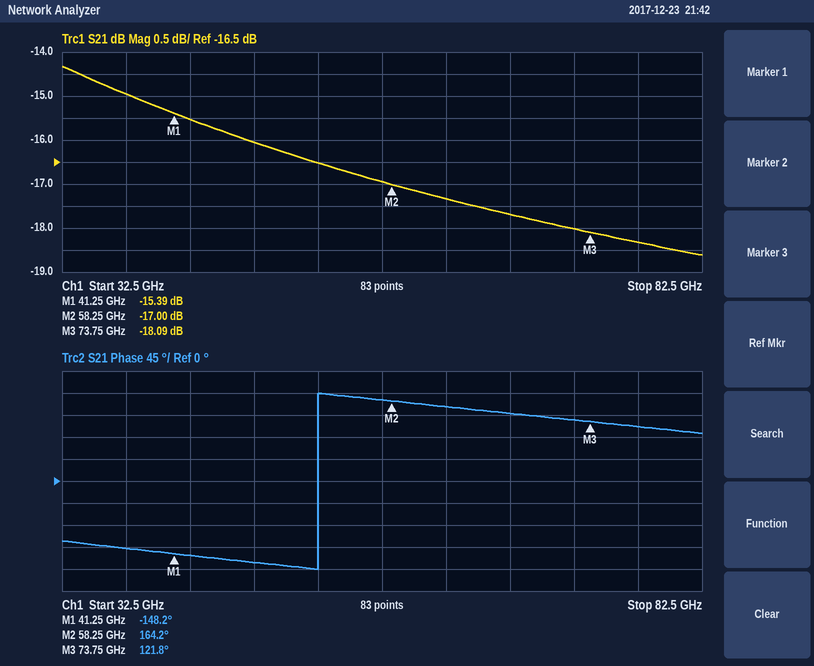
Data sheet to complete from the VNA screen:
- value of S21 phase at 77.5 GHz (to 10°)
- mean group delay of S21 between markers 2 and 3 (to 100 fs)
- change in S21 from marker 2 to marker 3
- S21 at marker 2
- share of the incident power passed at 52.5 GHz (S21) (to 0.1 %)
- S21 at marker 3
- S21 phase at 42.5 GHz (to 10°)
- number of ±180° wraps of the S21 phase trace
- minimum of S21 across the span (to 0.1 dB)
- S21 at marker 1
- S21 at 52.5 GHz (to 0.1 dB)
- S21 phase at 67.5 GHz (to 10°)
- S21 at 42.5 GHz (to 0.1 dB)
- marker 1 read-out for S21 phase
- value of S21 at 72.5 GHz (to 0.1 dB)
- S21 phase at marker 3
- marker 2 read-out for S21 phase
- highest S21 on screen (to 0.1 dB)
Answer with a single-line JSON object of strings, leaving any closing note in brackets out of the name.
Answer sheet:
{"value of S21 phase at 77.5 GHz": "110°", "mean group delay of S21 between markers 2 and 3": "7.6 ps", "change in S21 from marker 2 to marker 3": "-1.09 dB", "S21 at marker 2": "-17.00 dB", "share of the incident power passed at 52.5 GHz (S21)": "2.2 %", "S21 at marker 3": "-18.09 dB", "S21 phase at 42.5 GHz": "-150°", "number of ±180° wraps of the S21 phase trace": "1", "minimum of S21 across the span": "-18.6 dB", "S21 at marker 1": "-15.39 dB", "S21 at 52.5 GHz": "-16.5 dB", "S21 phase at 67.5 GHz": "140°", "S21 at 42.5 GHz": "-15.5 dB", "marker 1 read-out for S21 phase": "-148.2°", "value of S21 at 72.5 GHz": "-18.0 dB", "S21 phase at marker 3": "121.8°", "marker 2 read-out for S21 phase": "164.2°", "highest S21 on screen": "-14.3 dB"}
